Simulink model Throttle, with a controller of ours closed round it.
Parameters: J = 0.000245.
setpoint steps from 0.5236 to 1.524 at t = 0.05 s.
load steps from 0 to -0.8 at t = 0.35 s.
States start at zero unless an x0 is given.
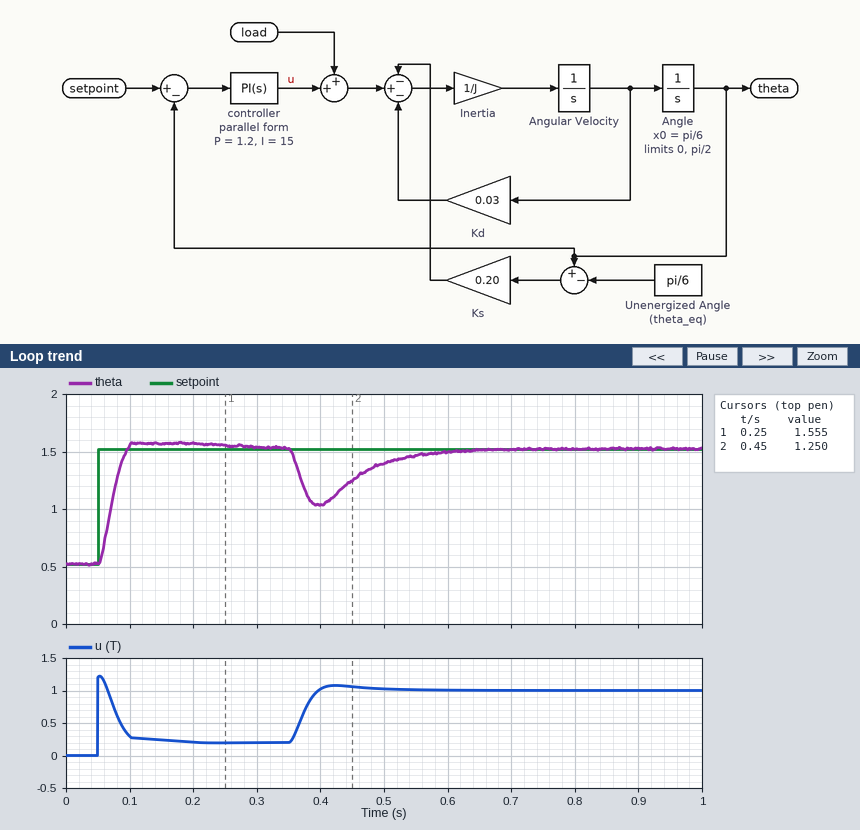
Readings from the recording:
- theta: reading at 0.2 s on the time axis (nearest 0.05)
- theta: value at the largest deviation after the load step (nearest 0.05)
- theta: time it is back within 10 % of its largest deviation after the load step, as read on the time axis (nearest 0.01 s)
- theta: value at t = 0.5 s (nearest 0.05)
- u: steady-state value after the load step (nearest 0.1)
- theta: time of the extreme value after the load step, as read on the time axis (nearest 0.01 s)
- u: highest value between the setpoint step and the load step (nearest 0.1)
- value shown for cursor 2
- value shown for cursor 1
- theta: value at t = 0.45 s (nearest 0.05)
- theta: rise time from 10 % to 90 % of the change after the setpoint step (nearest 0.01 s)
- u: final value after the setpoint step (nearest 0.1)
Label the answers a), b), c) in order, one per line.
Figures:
a) 1.55
b) 1.05
c) 0.56 s
d) 1.40
e) 1.0
f) 0.40 s
g) 1.2
h) 1.250
i) 1.555
j) 1.25
k) 0.03 s
l) 0.2
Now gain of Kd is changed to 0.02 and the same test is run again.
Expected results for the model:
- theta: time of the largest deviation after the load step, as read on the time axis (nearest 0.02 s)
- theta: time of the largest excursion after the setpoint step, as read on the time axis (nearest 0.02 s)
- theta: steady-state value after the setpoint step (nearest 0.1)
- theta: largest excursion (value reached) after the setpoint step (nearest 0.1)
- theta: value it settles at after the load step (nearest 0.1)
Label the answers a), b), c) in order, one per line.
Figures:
a) 0.40 s
b) 0.08 s
c) 1.5
d) 1.6
e) 1.5
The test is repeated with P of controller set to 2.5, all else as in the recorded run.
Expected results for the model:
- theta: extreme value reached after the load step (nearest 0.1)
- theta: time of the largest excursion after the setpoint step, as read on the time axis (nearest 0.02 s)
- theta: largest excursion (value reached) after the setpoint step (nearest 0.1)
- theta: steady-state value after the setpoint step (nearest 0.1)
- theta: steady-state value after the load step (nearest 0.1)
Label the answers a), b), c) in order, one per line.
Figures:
a) 1.2
b) 0.08 s
c) 1.6
d) 1.5
e) 1.5
